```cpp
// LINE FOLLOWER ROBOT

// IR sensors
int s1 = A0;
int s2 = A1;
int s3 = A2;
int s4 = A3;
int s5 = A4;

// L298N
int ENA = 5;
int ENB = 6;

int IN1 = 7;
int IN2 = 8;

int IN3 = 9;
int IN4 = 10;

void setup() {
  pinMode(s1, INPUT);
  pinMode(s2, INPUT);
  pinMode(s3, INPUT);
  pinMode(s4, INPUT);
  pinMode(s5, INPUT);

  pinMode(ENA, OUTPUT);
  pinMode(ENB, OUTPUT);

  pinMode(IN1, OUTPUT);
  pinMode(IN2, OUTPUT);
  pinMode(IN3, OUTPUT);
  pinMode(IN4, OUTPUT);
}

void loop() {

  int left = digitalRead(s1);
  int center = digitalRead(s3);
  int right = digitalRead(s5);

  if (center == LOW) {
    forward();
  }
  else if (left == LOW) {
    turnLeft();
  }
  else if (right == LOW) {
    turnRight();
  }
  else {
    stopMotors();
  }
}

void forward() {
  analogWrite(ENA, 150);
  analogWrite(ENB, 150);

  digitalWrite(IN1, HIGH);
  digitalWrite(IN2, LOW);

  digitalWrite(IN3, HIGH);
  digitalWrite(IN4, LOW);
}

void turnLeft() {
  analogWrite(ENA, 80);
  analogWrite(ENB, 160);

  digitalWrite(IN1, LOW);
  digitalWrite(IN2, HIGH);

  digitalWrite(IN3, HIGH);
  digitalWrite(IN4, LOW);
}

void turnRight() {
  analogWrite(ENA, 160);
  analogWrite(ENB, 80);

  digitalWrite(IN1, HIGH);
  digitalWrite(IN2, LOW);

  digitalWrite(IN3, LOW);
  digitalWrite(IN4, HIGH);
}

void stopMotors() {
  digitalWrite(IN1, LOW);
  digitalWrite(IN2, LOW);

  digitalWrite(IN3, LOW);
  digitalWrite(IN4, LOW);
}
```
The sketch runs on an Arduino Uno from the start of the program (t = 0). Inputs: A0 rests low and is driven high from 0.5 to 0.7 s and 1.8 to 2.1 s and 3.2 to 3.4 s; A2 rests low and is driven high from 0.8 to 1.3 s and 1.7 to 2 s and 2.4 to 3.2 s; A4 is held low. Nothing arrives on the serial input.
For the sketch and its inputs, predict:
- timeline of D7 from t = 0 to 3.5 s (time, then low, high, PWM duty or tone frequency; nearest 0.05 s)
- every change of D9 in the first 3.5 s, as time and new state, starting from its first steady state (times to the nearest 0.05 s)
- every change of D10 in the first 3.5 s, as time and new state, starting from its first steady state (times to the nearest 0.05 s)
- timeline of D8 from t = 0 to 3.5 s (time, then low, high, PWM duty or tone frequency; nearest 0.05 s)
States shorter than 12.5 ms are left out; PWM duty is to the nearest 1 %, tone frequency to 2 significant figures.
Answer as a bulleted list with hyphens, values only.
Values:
- 0 s high; 0.8 s low; 1.3 s high; 1.7 s low; 1.8 s high; 2.4 s low; 3.2 s high
- 0 s high; 1.8 s low; 2 s high
- 0 s low; 1.8 s high; 2 s low
- 0 s low; 0.8 s high; 1.3 s low; 1.7 s high; 1.8 s low; 2.4 s high; 3.2 s low
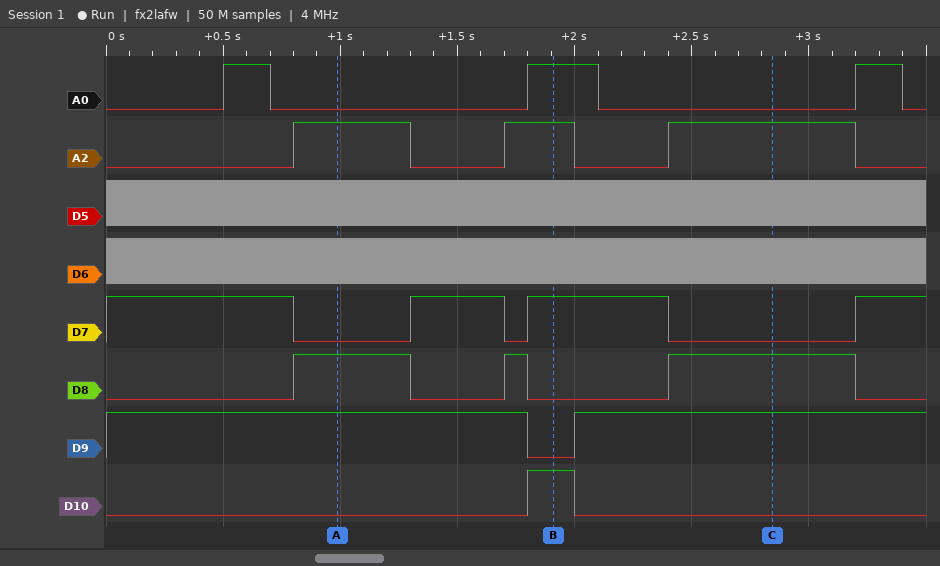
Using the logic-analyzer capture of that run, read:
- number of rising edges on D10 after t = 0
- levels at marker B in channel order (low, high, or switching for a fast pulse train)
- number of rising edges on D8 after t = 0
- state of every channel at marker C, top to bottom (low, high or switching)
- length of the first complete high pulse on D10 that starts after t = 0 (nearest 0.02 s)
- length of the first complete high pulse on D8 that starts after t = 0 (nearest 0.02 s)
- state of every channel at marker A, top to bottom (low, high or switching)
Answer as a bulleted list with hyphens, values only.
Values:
- 1
- A0 high, A2 high, D5 switching, D6 switching, D7 high, D8 low, D9 low, D10 high
- 3
- A0 low, A2 high, D5 switching, D6 switching, D7 low, D8 high, D9 high, D10 low
- 0.20 s
- 0.50 s
- A0 low, A2 high, D5 switching, D6 switching, D7 low, D8 high, D9 high, D10 low
